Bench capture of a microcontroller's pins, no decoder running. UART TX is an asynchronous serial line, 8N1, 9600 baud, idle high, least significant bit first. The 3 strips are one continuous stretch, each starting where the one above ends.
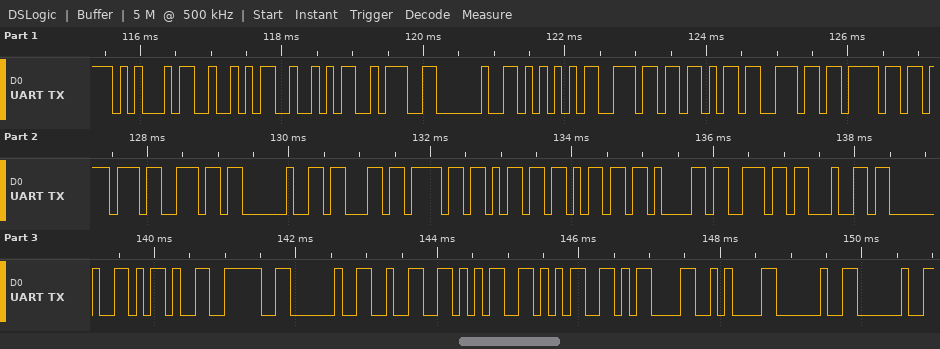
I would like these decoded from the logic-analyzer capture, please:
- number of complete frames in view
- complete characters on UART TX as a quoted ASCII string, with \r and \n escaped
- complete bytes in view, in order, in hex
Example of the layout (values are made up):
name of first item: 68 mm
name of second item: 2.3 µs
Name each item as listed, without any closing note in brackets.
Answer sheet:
number of complete frames in view: 31
complete characters on UART TX as a quoted ASCII string, with \r and \n escaped: "ERR: Unknown command -> 255\r\n  "
complete bytes in view, in order, in hex: 45 52 52 3A 20 55 6E 6B 6E 6F 77 6E 20 63 6F 6D 6D 61 6E 64 20 2D 3E 20 32 35 35 0D 0A 20 20
